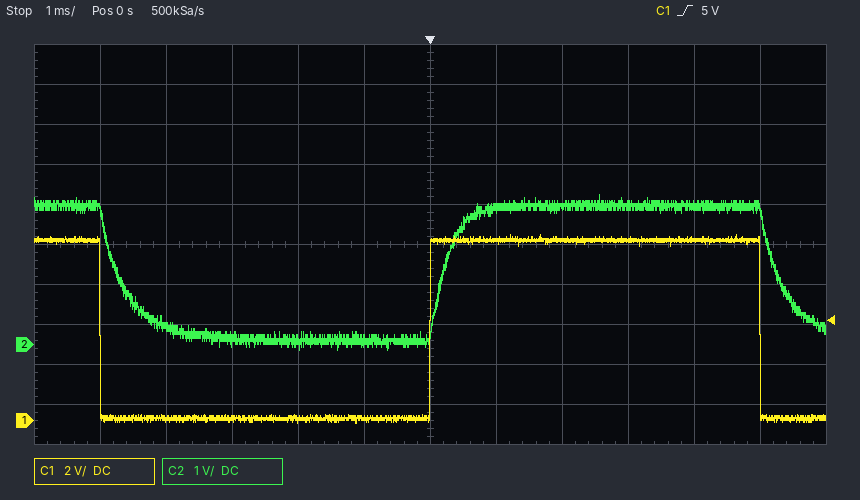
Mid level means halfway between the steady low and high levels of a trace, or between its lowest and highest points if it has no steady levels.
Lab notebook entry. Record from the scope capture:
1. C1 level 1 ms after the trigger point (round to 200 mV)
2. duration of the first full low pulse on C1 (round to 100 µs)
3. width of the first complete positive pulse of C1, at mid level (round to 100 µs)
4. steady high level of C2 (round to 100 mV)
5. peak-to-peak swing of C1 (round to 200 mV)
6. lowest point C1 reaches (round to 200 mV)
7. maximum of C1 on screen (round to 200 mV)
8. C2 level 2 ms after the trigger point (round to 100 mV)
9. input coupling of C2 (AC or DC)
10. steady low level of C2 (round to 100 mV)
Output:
9.0 V
5.0 ms
5.0 ms
3.5 V
9.4 V
-200 mV
9.2 V
3.4 V
DC
100 mV
